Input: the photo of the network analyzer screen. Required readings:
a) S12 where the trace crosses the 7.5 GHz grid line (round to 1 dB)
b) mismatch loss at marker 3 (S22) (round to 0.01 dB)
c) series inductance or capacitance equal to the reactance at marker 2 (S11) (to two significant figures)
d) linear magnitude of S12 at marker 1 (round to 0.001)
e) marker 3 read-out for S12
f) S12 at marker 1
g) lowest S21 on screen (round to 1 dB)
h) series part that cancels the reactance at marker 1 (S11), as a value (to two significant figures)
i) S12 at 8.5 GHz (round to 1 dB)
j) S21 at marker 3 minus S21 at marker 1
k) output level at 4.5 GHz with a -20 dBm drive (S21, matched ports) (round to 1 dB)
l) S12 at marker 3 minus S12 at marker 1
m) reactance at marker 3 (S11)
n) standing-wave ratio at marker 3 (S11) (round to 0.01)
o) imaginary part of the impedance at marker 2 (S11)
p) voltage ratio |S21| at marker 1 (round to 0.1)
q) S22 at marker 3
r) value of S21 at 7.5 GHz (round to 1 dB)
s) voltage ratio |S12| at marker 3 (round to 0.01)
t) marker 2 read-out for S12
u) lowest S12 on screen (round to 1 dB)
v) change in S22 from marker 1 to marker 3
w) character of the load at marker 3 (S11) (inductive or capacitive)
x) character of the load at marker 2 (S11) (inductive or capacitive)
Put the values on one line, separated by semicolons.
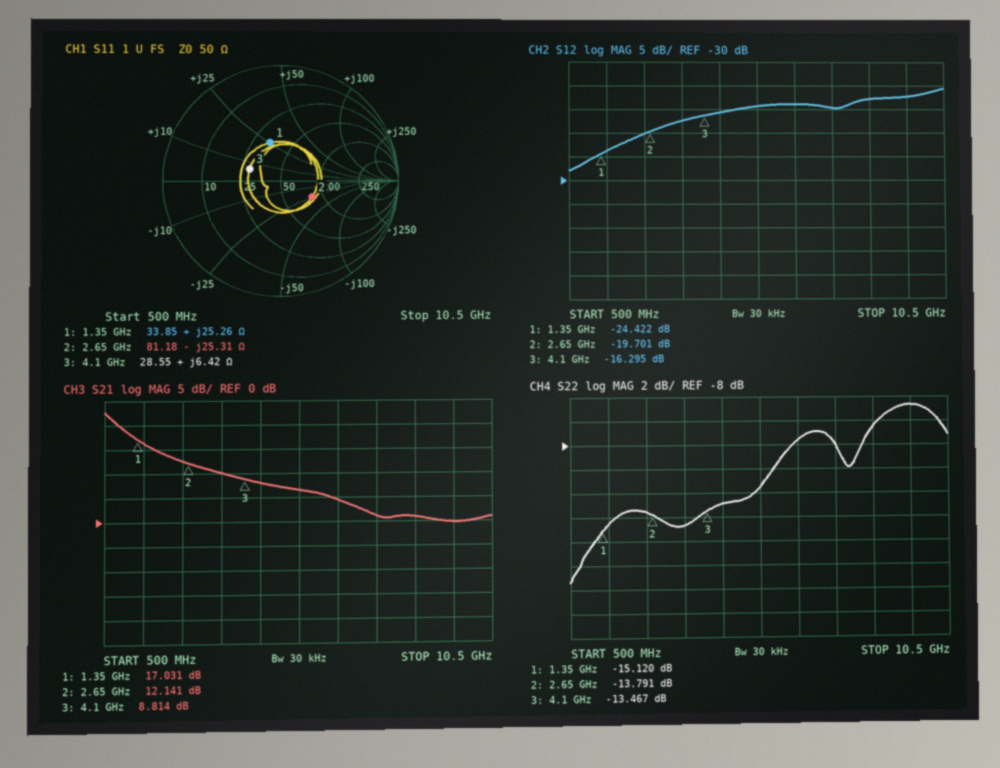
-15 dB; 0.20 dB; 2.4 pF; 0.060; -16.295 dB; -24.422 dB; 0 dB; 4.7 pF; -13 dB; -8.217 dB; -12 dBm; 8.127 dB; +6.42 Ω; 1.79; -25.31 Ω; 7.1; -13.467 dB; 1 dB; 0.15; -19.701 dB; -28 dB; 1.653 dB; inductive; capacitive
